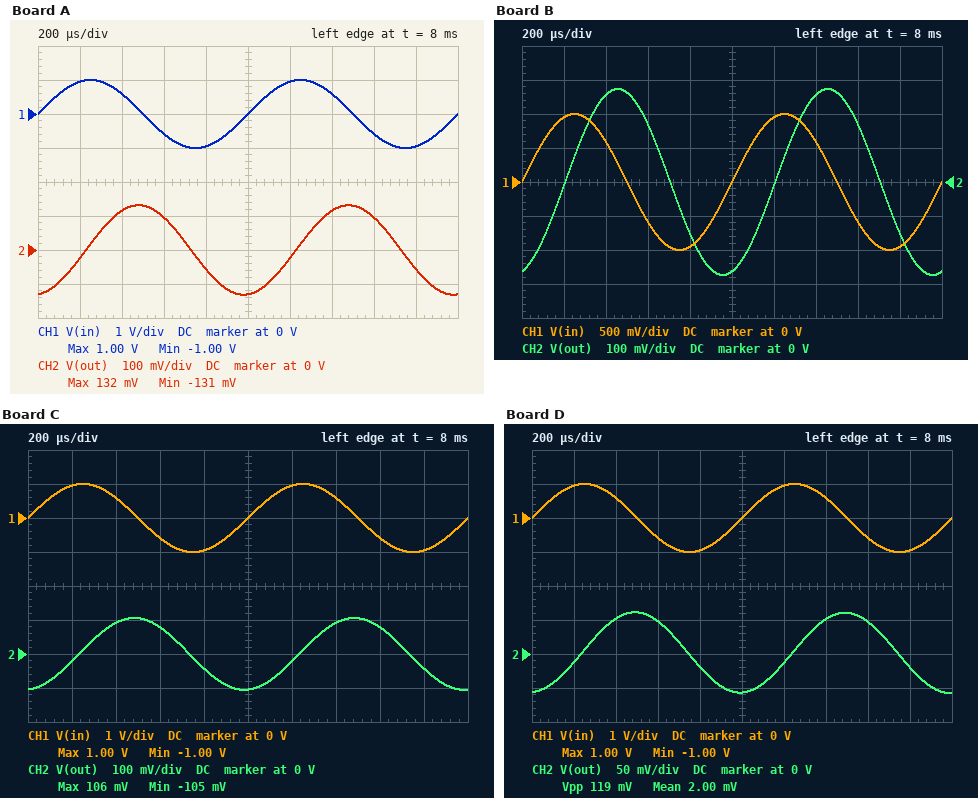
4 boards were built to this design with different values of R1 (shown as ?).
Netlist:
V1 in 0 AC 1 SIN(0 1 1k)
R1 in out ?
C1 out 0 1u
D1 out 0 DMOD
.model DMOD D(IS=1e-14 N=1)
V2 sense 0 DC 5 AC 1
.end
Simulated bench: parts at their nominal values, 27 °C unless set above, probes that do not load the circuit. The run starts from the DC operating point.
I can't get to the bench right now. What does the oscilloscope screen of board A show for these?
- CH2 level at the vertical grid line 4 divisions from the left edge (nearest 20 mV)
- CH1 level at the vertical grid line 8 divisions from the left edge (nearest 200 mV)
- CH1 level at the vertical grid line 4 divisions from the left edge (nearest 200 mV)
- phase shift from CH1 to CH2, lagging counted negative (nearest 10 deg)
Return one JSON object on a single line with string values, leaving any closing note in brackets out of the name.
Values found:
{"CH2 level at the vertical grid line 4 divisions from the left edge": "-60 mV", "CH1 level at the vertical grid line 8 divisions from the left edge": "-600 mV", "CH1 level at the vertical grid line 4 divisions from the left edge": "-1.0 V", "phase shift from CH1 to CH2, lagging counted negative": "-80 deg"}
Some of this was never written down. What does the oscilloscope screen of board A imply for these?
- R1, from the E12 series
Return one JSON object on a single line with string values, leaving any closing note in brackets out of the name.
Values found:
{"R1, from the E12 series": "1.2 kΩ"}
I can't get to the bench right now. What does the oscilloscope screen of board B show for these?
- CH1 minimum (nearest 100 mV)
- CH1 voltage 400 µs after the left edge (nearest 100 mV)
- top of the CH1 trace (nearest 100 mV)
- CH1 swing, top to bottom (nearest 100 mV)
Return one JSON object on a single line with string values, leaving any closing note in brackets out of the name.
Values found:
{"CH1 minimum": "-1.0 V", "CH1 voltage 400 µs after the left edge": "600 mV", "top of the CH1 trace": "1.0 V", "CH1 swing, top to bottom": "2.0 V"}
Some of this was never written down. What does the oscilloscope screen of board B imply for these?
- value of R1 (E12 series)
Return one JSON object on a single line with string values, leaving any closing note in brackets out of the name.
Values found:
{"value of R1": "560 Ω"}
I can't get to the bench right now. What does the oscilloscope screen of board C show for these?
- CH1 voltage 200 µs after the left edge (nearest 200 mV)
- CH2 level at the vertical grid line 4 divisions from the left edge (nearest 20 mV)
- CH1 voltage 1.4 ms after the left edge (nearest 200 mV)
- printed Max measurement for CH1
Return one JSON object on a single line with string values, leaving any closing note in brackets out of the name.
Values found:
{"CH1 voltage 200 µs after the left edge": "1.0 V", "CH2 level at the vertical grid line 4 divisions from the left edge": "-40 mV", "CH1 voltage 1.4 ms after the left edge": "600 mV", "printed Max measurement for CH1": "1.00 V"}
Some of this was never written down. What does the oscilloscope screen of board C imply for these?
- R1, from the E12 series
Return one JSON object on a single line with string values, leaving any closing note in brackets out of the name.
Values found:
{"R1, from the E12 series": "1.5 kΩ"}
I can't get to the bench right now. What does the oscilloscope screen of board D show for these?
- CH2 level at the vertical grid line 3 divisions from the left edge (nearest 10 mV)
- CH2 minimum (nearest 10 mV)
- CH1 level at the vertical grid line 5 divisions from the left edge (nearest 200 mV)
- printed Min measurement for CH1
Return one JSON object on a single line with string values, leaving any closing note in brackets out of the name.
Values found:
{"CH2 level at the vertical grid line 3 divisions from the left edge": "50 mV", "CH2 minimum": "-60 mV", "CH1 level at the vertical grid line 5 divisions from the left edge": "0 V", "printed Min measurement for CH1": "-1.00 V"}
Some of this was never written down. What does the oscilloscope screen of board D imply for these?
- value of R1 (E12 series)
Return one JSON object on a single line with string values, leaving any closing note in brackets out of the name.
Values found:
{"value of R1": "2.7 kΩ"}
